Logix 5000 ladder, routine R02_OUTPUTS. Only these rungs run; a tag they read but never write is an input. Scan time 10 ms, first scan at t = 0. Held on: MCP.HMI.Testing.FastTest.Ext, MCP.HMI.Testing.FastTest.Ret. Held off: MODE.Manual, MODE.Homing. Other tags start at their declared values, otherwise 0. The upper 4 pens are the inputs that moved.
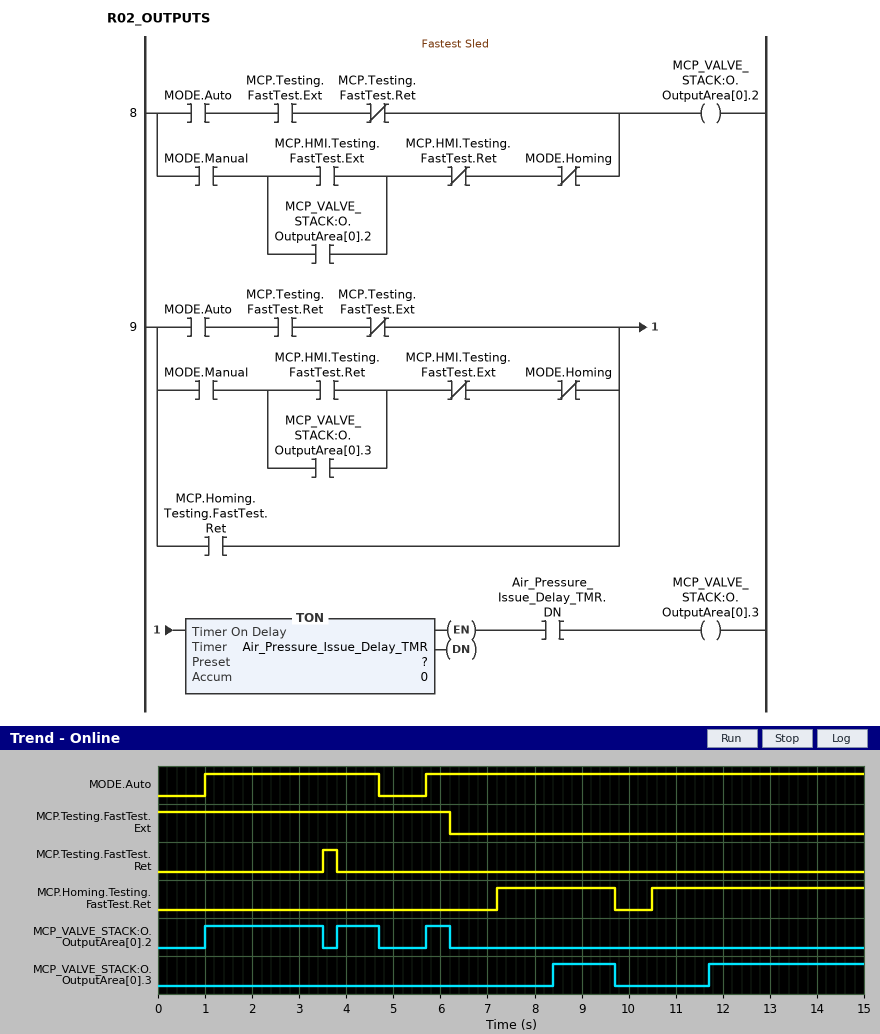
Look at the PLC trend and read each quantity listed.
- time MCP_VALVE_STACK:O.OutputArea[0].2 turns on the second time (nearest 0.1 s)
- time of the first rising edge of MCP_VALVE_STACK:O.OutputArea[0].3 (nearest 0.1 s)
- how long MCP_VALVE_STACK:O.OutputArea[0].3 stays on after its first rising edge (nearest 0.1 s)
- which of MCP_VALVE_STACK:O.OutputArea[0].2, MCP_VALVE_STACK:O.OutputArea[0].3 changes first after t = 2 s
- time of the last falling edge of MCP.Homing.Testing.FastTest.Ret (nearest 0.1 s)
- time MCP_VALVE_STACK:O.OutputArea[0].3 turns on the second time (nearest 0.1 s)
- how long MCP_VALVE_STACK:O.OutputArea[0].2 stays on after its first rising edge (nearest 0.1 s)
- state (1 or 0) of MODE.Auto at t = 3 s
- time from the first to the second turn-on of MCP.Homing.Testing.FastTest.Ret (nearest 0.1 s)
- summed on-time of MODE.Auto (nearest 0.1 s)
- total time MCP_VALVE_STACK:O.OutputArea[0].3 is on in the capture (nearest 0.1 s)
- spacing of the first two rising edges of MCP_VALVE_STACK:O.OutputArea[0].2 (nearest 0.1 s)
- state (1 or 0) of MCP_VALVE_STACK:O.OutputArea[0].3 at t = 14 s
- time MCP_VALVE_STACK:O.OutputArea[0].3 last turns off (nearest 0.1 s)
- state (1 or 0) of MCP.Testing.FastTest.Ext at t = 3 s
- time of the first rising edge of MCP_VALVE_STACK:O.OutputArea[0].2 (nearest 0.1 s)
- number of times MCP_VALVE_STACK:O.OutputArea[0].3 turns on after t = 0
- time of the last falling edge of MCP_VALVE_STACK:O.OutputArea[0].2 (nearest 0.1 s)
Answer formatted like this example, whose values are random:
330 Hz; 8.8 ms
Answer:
3.8 s; 8.4 s; 1.3 s; MCP_VALVE_STACK:O.OutputArea[0].2; 9.7 s; 11.7 s; 2.5 s; 1; 3.3 s; 13.0 s; 4.6 s; 2.8 s; 1; 9.7 s; 1; 1.0 s; 2; 6.2 s
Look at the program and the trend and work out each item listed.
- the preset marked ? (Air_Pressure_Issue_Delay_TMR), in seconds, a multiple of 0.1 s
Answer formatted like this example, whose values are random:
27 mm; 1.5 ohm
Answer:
1.2 s
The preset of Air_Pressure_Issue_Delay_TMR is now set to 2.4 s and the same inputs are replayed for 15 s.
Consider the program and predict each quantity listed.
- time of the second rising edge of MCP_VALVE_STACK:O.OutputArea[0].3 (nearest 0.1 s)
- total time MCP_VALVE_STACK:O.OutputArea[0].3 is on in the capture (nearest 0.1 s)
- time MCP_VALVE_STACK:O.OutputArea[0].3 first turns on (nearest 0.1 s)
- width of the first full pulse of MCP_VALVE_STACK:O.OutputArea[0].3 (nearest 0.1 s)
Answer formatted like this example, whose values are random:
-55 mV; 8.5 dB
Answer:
12.9 s; 2.2 s; 9.6 s; 0.1 s
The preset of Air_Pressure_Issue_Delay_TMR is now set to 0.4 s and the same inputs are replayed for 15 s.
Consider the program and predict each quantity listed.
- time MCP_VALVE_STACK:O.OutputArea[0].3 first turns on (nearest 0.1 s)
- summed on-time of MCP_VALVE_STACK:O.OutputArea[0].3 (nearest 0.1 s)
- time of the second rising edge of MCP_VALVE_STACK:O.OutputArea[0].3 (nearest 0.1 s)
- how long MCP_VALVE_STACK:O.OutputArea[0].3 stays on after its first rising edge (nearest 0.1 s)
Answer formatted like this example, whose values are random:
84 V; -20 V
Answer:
7.6 s; 6.2 s; 10.9 s; 2.1 s
